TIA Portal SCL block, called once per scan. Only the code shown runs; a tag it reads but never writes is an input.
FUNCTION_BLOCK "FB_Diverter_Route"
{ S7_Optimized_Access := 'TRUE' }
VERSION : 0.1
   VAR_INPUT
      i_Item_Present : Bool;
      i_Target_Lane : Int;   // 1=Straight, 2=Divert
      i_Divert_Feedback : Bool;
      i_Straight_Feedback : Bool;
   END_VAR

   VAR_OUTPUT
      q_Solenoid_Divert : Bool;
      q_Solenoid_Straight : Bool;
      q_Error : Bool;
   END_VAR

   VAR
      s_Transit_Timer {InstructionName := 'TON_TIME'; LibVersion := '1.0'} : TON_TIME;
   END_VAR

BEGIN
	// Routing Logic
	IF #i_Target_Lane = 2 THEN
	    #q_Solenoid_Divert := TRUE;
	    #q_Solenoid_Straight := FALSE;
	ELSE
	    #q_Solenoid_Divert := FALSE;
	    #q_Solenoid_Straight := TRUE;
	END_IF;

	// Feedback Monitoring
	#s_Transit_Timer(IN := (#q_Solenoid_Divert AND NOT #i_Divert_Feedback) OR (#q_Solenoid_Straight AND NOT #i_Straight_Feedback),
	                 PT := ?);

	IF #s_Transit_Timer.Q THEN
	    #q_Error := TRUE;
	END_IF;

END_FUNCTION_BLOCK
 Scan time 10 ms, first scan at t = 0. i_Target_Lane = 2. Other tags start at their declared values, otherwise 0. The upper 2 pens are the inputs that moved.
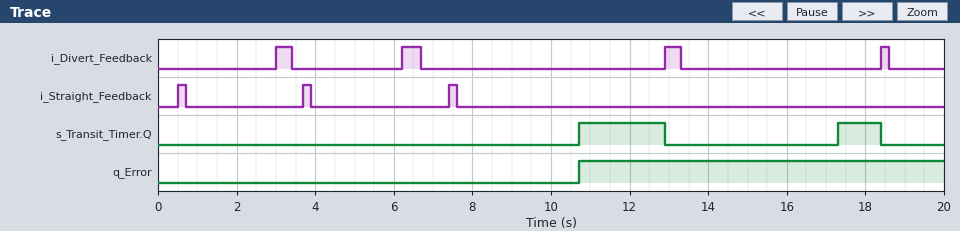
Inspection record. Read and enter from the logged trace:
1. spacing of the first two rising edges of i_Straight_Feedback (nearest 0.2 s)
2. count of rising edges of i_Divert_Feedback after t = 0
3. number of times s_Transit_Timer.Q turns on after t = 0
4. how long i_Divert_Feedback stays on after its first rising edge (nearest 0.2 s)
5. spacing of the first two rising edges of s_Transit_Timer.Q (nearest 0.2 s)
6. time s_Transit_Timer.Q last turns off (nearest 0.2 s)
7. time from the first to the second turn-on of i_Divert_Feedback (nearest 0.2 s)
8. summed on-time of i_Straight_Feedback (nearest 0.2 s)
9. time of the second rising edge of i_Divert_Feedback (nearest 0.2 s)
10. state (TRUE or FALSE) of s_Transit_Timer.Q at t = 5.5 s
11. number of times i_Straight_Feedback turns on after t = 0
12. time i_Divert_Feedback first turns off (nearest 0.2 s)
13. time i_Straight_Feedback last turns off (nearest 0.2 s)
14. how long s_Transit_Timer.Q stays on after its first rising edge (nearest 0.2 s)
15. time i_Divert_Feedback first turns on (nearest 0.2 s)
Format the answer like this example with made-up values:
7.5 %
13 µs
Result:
3.2 s
4
2
0.4 s
6.6 s
18.4 s
3.2 s
0.6 s
6.2 s
FALSE
3
3.4 s
7.6 s
2.2 s
3.0 s
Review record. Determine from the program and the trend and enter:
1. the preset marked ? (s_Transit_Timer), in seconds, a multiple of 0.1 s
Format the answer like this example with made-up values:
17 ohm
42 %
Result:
4.0 s
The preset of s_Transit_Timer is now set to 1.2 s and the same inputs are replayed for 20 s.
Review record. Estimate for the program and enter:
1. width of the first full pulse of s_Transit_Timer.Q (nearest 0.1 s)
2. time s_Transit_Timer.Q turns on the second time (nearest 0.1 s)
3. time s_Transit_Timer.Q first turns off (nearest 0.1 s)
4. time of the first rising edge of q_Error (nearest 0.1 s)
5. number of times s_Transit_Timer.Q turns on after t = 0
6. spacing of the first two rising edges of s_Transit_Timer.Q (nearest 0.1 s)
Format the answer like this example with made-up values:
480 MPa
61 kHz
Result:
1.8 s
4.6 s
3.0 s
1.2 s
5
3.4 s
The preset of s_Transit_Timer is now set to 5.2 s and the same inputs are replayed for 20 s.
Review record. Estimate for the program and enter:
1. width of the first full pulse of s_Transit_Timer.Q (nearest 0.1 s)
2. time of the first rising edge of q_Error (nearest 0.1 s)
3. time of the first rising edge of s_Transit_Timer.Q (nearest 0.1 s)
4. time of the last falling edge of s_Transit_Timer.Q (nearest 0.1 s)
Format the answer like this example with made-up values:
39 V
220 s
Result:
1.0 s
11.9 s
11.9 s
12.9 s
